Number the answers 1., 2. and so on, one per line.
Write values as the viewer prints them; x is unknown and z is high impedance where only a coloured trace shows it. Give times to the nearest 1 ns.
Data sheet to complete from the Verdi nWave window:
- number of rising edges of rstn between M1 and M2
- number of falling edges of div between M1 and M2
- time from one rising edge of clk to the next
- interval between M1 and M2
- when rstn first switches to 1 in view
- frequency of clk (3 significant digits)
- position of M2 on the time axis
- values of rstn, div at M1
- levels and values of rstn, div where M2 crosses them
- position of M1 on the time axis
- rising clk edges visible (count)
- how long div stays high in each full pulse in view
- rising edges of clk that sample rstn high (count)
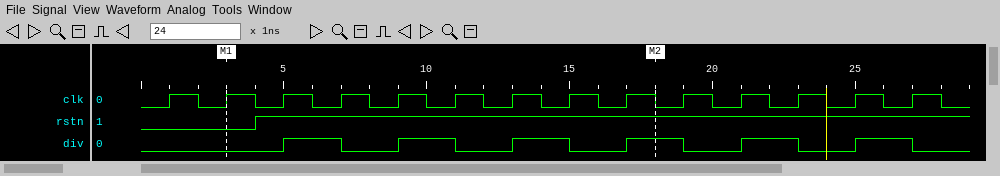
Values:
1. 1
2. 3
3. 2 ns
4. 15 ns
5. 4 ns
6. 500 MHz
7. 18 ns
8. rstn=0, div=0
9. rstn=1, div=1
10. 3 ns
11. 14
12. 2 ns, 2 ns, 2 ns, 2 ns, 2 ns, 2 ns
13. 12
